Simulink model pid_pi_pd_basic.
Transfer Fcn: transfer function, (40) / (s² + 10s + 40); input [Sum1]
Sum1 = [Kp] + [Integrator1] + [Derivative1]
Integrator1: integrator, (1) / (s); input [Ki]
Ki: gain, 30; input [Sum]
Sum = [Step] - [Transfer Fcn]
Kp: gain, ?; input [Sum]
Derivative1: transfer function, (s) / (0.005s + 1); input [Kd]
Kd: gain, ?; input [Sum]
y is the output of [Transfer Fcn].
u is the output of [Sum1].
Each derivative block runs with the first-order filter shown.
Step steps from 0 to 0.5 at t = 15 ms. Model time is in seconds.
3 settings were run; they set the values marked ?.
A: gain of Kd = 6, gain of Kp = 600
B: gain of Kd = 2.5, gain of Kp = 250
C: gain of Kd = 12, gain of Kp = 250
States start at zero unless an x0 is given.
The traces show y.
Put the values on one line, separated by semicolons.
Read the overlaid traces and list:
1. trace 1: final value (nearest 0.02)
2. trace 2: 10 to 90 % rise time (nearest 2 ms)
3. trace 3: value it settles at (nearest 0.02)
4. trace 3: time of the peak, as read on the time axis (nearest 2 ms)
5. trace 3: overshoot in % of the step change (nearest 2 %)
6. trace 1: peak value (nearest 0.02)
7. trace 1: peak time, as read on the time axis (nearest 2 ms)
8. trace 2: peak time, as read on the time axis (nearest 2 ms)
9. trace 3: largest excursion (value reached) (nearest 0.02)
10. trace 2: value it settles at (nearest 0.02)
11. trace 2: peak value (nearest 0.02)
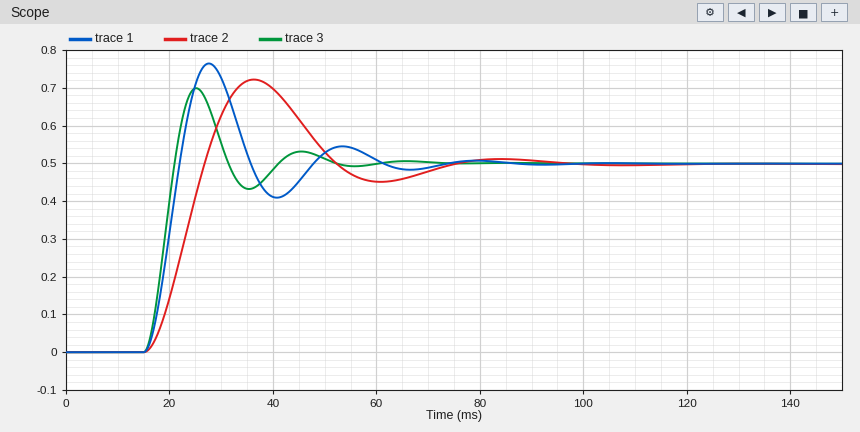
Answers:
0.50; 8 ms; 0.50; 26 ms; 40 %; 0.76; 28 ms; 36 ms; 0.70; 0.50; 0.72
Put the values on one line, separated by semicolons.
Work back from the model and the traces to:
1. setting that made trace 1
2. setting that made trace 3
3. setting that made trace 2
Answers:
A; C; B
